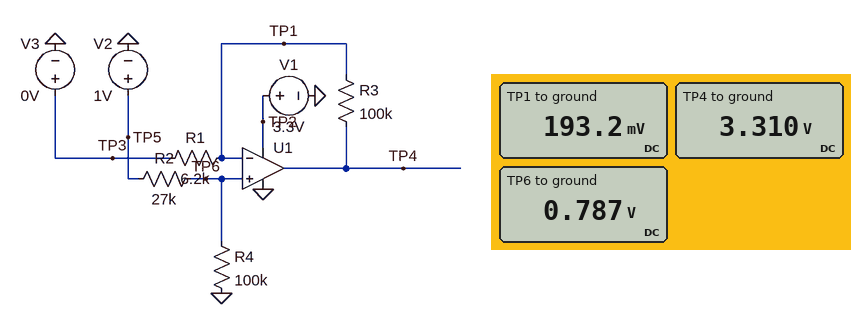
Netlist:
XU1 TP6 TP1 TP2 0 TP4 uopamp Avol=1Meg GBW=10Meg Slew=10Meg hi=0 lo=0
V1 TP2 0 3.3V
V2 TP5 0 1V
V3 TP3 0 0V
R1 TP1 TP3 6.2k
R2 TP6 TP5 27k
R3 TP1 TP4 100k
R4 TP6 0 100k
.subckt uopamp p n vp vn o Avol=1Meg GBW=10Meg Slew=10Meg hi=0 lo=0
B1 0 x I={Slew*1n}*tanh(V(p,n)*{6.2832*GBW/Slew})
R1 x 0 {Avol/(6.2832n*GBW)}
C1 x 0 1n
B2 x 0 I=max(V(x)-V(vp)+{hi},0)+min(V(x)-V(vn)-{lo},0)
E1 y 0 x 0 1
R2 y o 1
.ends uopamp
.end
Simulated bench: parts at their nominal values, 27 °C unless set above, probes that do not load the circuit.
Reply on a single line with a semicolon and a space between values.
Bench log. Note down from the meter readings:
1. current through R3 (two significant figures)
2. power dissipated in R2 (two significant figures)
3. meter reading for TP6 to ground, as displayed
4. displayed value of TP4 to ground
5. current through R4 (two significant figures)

31 µA; 1.7 µW; 0.787 V; 3.310 V; 7.9 µA
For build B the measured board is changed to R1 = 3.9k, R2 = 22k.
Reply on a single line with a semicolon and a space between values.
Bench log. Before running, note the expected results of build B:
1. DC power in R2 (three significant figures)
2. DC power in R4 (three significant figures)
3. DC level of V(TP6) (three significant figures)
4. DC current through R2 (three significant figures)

1.48 µW; 6.72 µW; 820 mV; 8.20 µA
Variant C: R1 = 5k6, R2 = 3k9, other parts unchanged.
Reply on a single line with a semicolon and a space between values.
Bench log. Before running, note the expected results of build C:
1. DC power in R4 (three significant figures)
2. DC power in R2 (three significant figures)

9.26 µW; 361 nW
